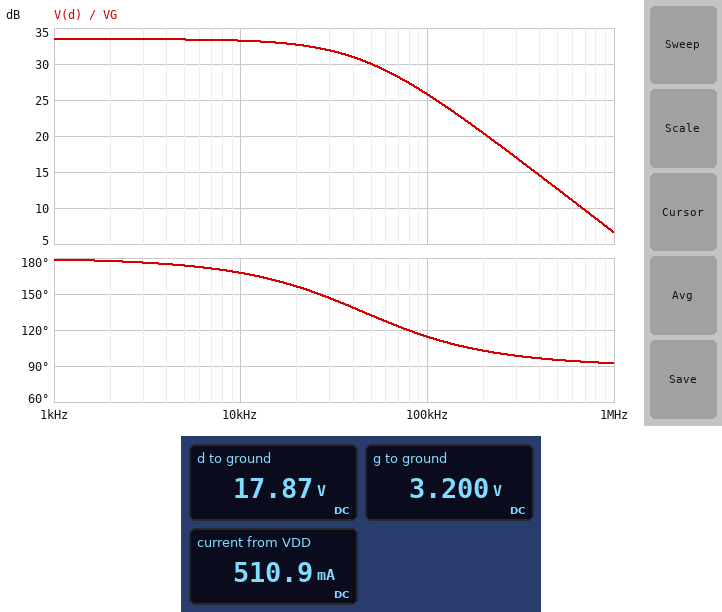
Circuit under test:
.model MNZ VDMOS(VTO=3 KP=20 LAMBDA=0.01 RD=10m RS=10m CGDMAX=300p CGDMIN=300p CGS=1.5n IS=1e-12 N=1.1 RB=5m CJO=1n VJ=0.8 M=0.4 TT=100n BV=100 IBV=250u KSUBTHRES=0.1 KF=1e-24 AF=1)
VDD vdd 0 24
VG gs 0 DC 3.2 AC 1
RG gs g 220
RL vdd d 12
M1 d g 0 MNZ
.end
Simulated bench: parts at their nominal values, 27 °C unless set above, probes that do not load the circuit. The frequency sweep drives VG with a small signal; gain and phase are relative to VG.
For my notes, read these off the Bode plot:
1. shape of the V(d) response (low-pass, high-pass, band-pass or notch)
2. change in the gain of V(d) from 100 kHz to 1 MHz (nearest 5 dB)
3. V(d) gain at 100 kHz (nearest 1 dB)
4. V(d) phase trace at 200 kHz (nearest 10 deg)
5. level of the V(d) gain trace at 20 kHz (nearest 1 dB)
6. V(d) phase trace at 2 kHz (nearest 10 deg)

low-pass
-20 dB
26 dB
100 deg
33 dB
180 deg
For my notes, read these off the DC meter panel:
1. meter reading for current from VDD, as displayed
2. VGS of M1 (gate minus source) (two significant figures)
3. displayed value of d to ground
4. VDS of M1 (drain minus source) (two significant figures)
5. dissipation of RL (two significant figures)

510.9 mA
3.2 V
17.87 V
18 V
3.1 W
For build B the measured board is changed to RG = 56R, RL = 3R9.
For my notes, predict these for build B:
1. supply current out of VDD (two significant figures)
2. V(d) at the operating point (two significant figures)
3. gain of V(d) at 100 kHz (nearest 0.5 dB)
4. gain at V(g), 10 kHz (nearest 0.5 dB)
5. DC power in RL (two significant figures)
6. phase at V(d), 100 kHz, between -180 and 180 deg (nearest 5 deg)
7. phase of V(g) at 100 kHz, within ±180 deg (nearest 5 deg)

530 mA
22 V
24.0 dB
0 dB
1.1 W
165 deg
-15 deg
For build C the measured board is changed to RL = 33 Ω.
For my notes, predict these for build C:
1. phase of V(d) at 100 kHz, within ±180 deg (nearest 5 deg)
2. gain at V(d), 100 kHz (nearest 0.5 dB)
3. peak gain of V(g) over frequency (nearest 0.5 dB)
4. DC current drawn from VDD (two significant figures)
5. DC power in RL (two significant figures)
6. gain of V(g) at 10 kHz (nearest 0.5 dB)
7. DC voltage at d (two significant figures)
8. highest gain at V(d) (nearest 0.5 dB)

100 deg
27.0 dB
0 dB
470 mA
7.3 W
-1.0 dB
8.4 V
41.0 dB
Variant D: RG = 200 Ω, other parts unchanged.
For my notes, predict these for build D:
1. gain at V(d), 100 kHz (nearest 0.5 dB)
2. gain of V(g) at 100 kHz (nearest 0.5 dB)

26.5 dB
-7.0 dB
